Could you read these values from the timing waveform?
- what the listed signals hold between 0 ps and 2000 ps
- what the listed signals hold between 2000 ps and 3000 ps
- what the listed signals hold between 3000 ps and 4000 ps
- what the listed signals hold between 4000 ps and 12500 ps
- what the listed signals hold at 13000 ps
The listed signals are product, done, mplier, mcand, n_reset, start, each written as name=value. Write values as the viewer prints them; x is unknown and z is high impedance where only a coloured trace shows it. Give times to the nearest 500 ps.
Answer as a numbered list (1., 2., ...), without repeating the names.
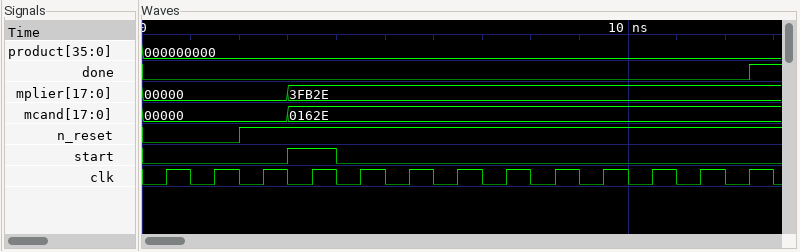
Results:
1. product=000000000, done=0, mplier=00000, mcand=00000, n_reset=0, start=0
2. product=000000000, done=0, mplier=00000, mcand=00000, n_reset=1, start=0
3. product=000000000, done=0, mplier=3FB2E, mcand=0162E, n_reset=1, start=1
4. product=000000000, done=0, mplier=3FB2E, mcand=0162E, n_reset=1, start=0
5. product=000000000, done=1, mplier=3FB2E, mcand=0162E, n_reset=1, start=0
